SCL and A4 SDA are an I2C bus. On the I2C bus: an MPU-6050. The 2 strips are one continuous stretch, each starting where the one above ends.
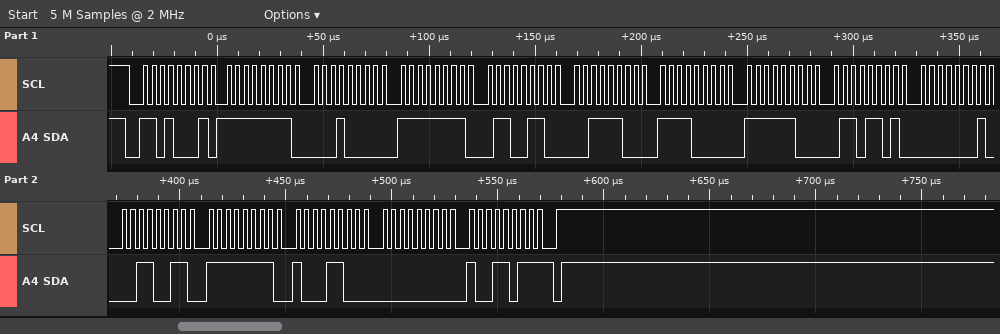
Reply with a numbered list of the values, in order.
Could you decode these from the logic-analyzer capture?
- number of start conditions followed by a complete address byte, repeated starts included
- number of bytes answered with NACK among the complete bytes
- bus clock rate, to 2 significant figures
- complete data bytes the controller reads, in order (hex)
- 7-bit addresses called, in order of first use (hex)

1. 1
2. 1
3. 250 kHz
4. FF 10 FF 66 3C F0 FC 6D 01 33 FF 8C 00 9B
5. 0x68
